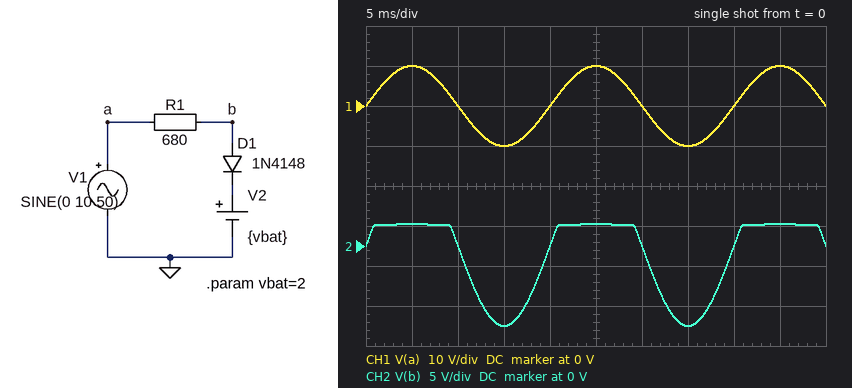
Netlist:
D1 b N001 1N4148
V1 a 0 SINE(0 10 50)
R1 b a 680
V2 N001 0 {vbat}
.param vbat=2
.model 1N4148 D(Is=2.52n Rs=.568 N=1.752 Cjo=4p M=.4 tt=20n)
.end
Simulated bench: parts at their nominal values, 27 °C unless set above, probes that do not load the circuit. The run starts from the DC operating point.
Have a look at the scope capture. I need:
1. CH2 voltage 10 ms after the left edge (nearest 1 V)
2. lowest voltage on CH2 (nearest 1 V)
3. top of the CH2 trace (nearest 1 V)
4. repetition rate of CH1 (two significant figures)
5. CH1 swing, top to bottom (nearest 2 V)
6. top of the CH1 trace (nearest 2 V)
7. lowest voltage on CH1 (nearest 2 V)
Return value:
0 V
-10 V
3 V
50 Hz
20 V
10 V
-10 V
